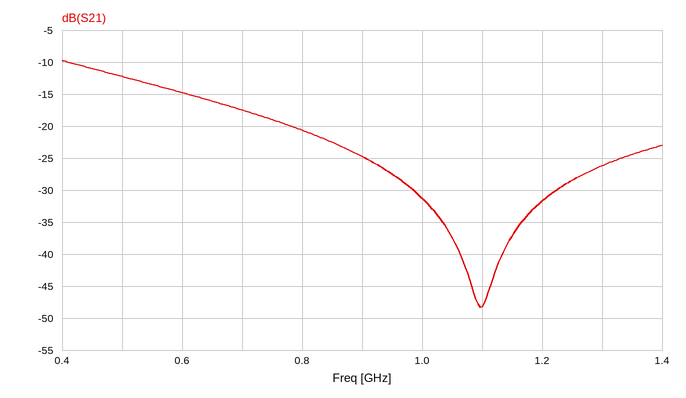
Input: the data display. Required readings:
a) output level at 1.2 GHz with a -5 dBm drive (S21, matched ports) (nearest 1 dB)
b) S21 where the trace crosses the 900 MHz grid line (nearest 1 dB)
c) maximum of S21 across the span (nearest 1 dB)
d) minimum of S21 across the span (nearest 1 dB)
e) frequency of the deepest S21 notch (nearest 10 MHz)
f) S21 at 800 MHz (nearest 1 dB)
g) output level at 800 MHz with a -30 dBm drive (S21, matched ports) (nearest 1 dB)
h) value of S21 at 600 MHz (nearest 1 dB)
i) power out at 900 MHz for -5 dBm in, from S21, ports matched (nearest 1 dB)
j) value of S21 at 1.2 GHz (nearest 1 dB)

-37 dBm
-25 dB
-10 dB
-48 dB
1.10 GHz
-21 dB
-51 dBm
-15 dB
-30 dBm
-32 dB
